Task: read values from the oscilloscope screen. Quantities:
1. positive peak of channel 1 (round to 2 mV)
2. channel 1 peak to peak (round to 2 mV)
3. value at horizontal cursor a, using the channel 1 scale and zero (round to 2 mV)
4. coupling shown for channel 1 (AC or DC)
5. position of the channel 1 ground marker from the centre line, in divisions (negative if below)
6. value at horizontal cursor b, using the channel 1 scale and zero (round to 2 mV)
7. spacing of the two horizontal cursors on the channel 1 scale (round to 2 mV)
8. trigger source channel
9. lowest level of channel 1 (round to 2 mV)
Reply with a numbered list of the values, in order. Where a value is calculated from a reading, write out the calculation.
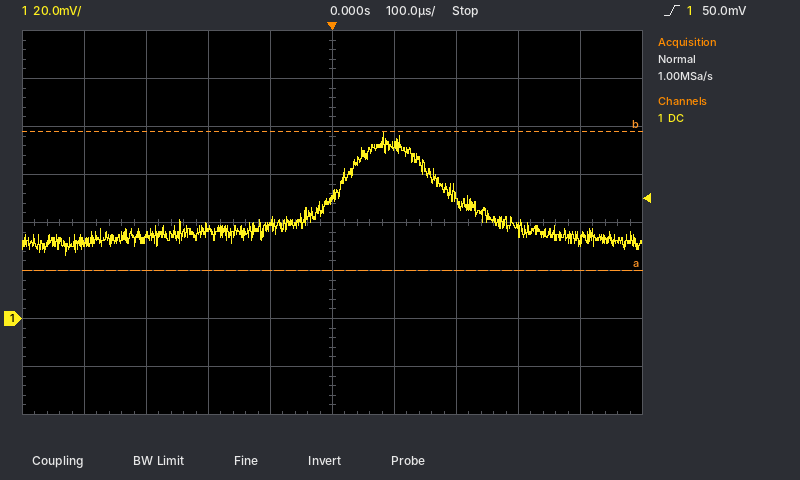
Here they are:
1. 78 mV
2. 78 mV − (26 mV) = 52 mV
3. 20 mV
4. DC
5. -2.0 div
6. 78 mV
7. 58 mV
8. channel 1
9. 26 mV
